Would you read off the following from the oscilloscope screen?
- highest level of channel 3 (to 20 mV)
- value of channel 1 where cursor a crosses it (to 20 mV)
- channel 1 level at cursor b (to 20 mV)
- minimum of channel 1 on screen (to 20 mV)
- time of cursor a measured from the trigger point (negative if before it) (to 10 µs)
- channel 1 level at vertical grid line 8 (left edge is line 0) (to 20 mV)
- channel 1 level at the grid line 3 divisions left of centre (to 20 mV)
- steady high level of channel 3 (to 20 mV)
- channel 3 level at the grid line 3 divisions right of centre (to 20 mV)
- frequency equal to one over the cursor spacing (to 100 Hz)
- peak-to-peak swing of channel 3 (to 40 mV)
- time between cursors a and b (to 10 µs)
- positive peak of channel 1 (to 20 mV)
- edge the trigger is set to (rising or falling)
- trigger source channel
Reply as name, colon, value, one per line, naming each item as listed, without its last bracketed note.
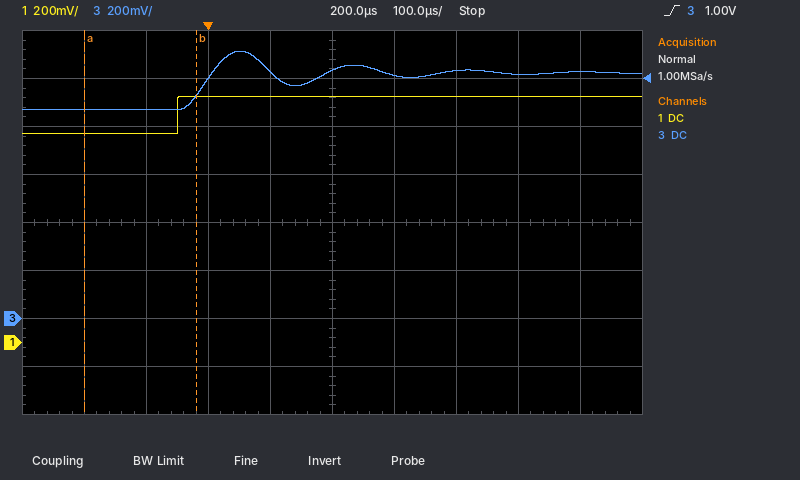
highest level of channel 3: 1.12 V
value of channel 1 where cursor a crosses it: 880 mV
channel 1 level at cursor b: 1.02 V
minimum of channel 1 on screen: 880 mV
time of cursor a measured from the trigger point (negative if before it): -200 µs
channel 1 level at vertical grid line 8 (left edge is line 0): 1.02 V
channel 1 level at the grid line 3 divisions left of centre: 880 mV
steady high level of channel 3: 1.02 V
channel 3 level at the grid line 3 divisions right of centre: 1.02 V
frequency equal to one over the cursor spacing: 5.6 kHz
peak-to-peak swing of channel 3: 240 mV
time between cursors a and b: 180 µs
positive peak of channel 1: 1.02 V
edge the trigger is set to: rising
trigger source channel: channel 3
